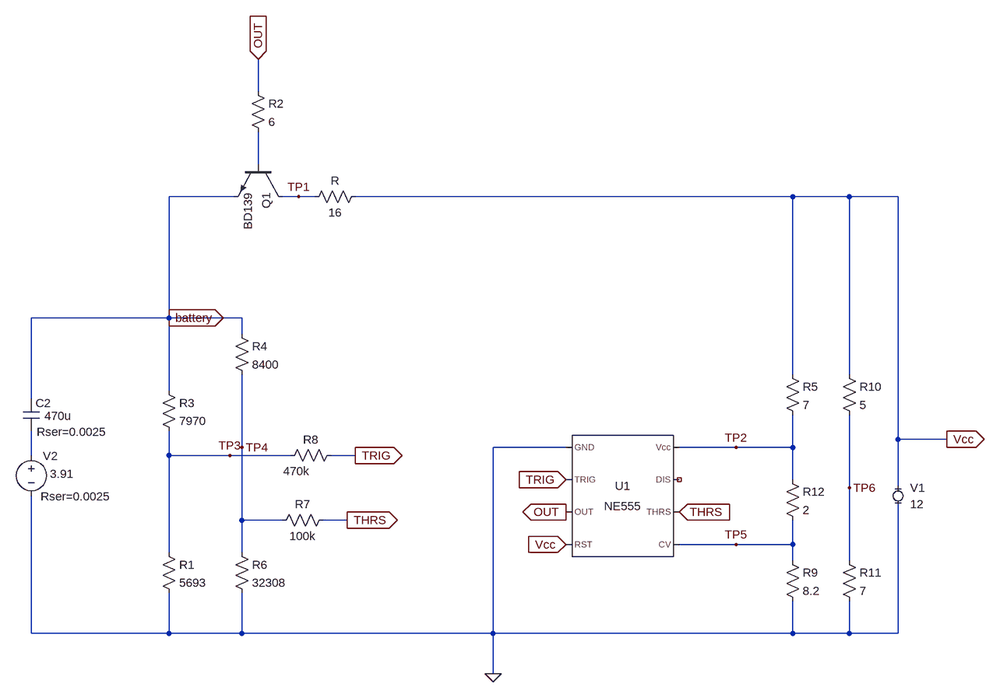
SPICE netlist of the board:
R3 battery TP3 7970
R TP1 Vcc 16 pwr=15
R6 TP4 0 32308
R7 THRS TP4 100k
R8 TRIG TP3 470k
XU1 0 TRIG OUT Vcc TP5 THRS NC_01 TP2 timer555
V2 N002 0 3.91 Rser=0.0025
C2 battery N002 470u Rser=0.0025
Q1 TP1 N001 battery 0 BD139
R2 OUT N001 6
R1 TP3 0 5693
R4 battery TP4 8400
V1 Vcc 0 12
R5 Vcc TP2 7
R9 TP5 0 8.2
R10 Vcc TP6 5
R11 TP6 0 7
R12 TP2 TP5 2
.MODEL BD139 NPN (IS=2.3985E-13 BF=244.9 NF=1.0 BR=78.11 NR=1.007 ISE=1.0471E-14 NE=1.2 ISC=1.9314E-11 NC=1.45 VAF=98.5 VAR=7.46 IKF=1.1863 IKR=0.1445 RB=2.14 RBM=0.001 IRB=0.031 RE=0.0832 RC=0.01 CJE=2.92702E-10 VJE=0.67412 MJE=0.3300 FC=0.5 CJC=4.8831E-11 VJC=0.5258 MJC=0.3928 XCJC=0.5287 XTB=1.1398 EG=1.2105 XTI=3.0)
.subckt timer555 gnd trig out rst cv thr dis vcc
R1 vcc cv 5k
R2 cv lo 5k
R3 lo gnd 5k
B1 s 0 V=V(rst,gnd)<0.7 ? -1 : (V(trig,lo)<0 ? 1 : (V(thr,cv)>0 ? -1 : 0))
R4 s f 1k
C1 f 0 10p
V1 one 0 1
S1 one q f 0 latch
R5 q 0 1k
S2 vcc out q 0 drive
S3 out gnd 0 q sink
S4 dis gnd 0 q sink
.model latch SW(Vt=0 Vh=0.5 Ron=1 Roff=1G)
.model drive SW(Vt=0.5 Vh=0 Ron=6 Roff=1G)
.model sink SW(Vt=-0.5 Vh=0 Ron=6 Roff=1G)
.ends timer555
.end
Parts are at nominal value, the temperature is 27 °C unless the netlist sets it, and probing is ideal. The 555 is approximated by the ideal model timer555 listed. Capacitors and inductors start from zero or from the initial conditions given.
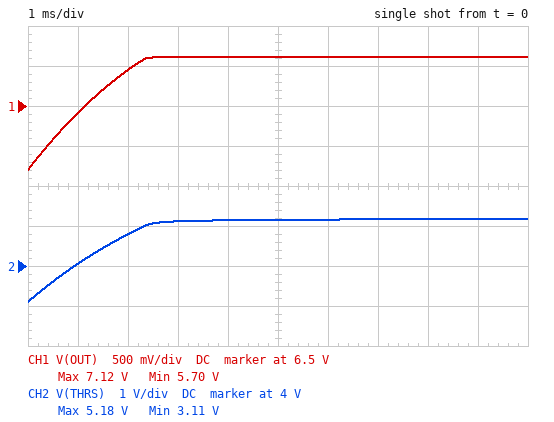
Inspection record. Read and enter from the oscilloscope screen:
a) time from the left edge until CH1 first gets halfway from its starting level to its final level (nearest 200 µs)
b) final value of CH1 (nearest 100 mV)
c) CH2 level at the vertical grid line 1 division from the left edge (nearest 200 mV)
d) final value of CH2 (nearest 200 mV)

1.0 ms
7.1 V
4.0 V
5.2 V
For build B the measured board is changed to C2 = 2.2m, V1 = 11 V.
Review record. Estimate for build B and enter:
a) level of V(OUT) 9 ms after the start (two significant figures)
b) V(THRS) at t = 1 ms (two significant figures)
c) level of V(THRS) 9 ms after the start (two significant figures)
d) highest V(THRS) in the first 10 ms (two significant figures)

6.5 V
3.3 V
4.5 V
4.6 V
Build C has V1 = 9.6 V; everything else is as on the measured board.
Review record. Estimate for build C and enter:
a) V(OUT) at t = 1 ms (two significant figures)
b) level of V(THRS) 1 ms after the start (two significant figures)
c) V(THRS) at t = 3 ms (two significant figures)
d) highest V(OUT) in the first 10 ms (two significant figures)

5.6 V
3.7 V
4.0 V
5.7 V
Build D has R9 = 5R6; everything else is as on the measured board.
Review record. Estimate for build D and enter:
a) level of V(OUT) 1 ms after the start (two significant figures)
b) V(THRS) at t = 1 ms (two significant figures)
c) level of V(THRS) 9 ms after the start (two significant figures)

6.0 V
4.0 V
4.5 V
